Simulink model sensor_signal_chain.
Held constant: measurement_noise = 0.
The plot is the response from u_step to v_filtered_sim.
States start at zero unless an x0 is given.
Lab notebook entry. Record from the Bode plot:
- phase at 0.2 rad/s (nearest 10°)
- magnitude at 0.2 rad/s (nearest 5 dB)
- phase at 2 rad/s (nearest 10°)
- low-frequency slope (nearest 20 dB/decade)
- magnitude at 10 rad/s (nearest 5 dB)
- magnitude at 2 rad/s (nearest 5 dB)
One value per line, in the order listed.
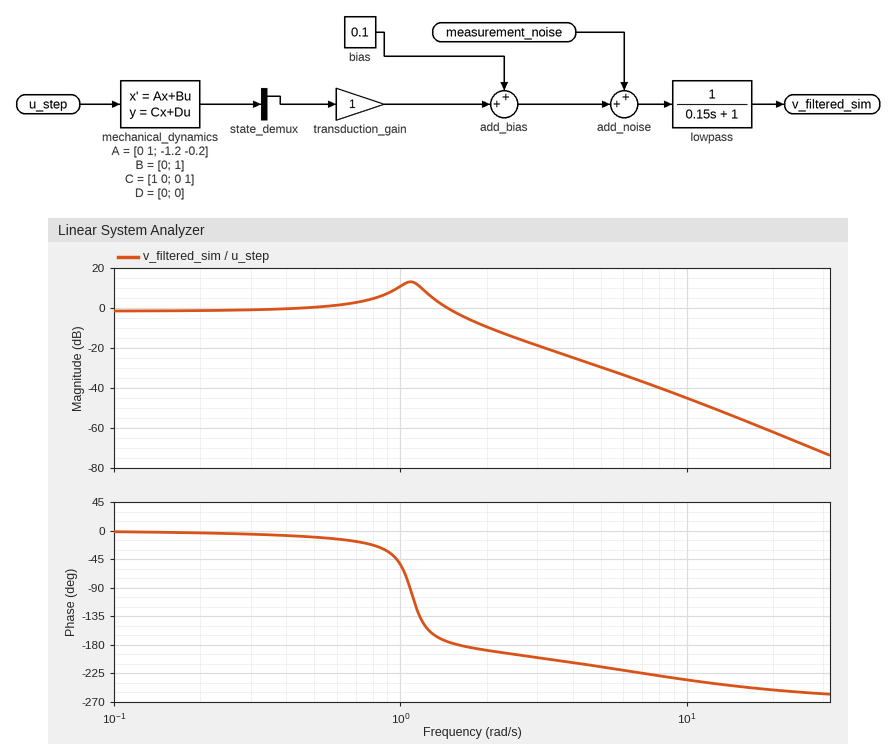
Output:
0°
0 dB
-190°
0 dB/decade
-45 dB
-10 dB
